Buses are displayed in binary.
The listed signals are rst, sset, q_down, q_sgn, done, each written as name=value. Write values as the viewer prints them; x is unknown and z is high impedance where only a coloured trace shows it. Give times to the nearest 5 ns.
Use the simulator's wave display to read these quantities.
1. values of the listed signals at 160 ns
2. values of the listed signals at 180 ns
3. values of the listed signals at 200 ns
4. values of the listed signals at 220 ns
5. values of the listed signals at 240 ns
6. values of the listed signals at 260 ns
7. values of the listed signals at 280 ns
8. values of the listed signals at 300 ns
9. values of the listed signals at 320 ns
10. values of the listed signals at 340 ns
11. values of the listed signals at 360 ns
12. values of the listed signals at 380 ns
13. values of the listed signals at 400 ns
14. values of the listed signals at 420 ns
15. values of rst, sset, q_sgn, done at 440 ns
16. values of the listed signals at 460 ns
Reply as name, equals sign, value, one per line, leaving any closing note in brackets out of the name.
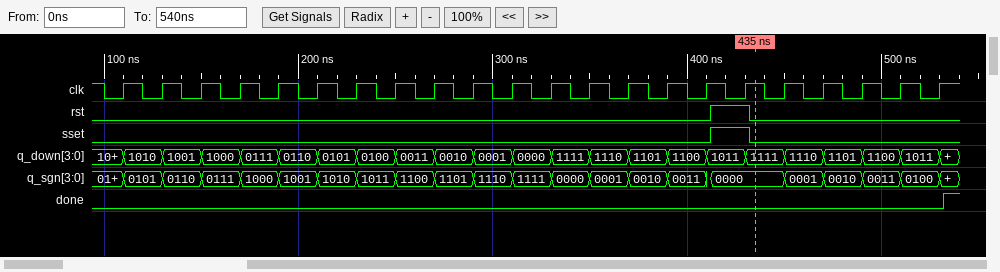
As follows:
values of the listed signals at 160 ns = rst=0, sset=0, q_down=1000, q_sgn=0111, done=0
values of the listed signals at 180 ns = rst=0, sset=0, q_down=0111, q_sgn=1000, done=0
values of the listed signals at 200 ns = rst=0, sset=0, q_down=0110, q_sgn=1001, done=0
values of the listed signals at 220 ns = rst=0, sset=0, q_down=0101, q_sgn=1010, done=0
values of the listed signals at 240 ns = rst=0, sset=0, q_down=0100, q_sgn=1011, done=0
values of the listed signals at 260 ns = rst=0, sset=0, q_down=0011, q_sgn=1100, done=0
values of the listed signals at 280 ns = rst=0, sset=0, q_down=0010, q_sgn=1101, done=0
values of the listed signals at 300 ns = rst=0, sset=0, q_down=0001, q_sgn=1110, done=0
values of the listed signals at 320 ns = rst=0, sset=0, q_down=0000, q_sgn=1111, done=0
values of the listed signals at 340 ns = rst=0, sset=0, q_down=1111, q_sgn=0000, done=0
values of the listed signals at 360 ns = rst=0, sset=0, q_down=1110, q_sgn=0001, done=0
values of the listed signals at 380 ns = rst=0, sset=0, q_down=1101, q_sgn=0010, done=0
values of the listed signals at 400 ns = rst=0, sset=0, q_down=1100, q_sgn=0011, done=0
values of the listed signals at 420 ns = rst=1, sset=1, q_down=1011, q_sgn=0000, done=0
values of rst, sset, q_sgn, done at 440 ns = rst=0, sset=0, q_sgn=0000, done=0
values of the listed signals at 460 ns = rst=0, sset=0, q_down=1110, q_sgn=0001, done=0
